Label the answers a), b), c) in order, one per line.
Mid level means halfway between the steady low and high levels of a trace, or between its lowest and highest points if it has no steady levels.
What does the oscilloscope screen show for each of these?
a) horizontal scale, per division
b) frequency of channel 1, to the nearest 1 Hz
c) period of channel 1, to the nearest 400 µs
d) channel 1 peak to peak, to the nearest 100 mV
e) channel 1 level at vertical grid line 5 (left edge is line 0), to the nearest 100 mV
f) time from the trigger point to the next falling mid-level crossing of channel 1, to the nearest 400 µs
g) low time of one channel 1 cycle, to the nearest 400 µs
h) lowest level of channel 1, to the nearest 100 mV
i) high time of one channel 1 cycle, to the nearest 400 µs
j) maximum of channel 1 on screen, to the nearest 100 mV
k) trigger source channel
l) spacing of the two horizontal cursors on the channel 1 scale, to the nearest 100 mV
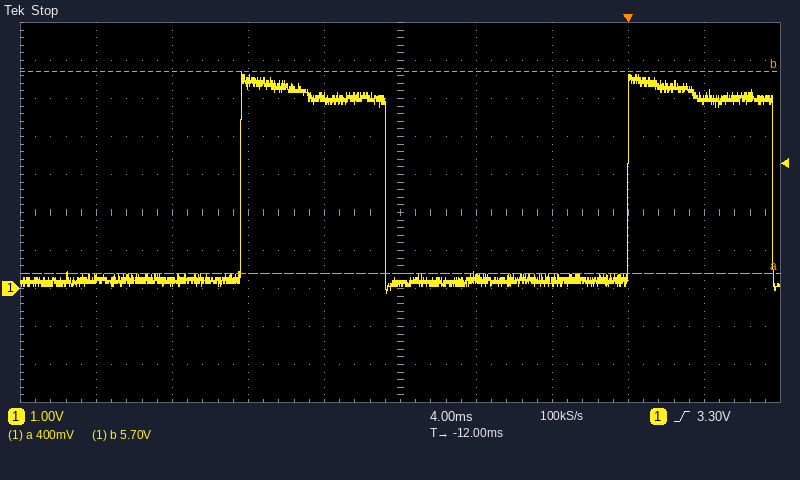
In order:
a) 4 ms
b) 49 Hz
c) 20.4 ms
d) 5.8 V
e) 100 mV
f) 7.6 ms
g) 12.8 ms
h) -100 mV
i) 7.6 ms
j) 5.7 V
k) channel 1
l) 5.3 V
